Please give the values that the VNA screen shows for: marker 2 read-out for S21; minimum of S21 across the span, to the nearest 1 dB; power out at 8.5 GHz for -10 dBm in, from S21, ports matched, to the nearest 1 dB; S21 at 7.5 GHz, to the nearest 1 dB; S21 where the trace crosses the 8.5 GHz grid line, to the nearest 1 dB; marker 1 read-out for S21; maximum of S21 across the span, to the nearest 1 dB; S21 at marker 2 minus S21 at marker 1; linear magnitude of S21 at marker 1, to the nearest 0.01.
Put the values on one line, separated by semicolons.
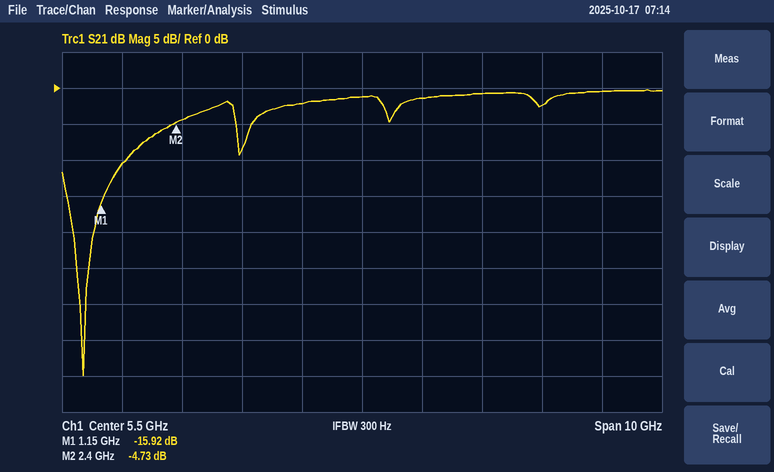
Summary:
-4.73 dB; -40 dB; -12 dBm; -1 dB; -2 dB; -15.92 dB; 0 dB; 11.19 dB; 0.16
